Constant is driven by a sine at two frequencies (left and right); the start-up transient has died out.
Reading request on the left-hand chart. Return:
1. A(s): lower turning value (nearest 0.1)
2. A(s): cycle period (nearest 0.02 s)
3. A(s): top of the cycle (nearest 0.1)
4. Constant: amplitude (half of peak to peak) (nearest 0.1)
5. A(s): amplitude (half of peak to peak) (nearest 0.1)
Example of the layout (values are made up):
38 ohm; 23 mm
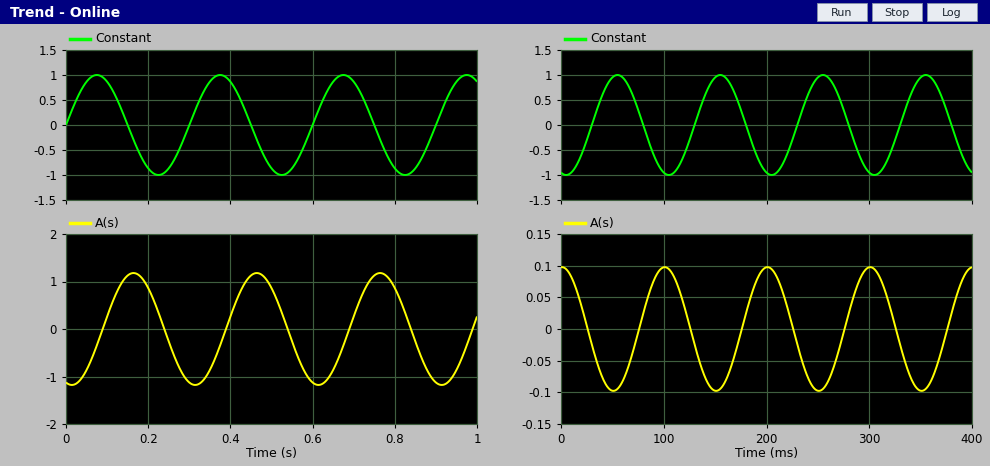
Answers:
-1.2; 0.30 s; 1.2; 1.0; 1.2
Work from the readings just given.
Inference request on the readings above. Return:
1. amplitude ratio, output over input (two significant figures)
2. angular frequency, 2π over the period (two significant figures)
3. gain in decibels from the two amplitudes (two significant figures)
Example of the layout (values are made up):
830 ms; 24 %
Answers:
1.2; 21 rad/s; 1.6 dB
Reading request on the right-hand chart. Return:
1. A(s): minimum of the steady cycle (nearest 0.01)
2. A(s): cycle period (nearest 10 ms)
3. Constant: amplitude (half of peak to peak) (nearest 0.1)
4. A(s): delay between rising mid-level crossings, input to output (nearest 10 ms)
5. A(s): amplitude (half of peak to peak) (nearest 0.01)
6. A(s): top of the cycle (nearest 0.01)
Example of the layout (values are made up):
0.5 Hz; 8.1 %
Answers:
-0.10; 100 ms; 1.0; 50 ms; 0.10; 0.10
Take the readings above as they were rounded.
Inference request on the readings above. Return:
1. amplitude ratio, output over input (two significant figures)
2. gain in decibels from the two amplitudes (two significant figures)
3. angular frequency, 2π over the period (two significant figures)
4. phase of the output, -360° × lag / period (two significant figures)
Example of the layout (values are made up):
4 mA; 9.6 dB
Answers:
0.10; -20 dB; 0.063 rad/ms; -180°
